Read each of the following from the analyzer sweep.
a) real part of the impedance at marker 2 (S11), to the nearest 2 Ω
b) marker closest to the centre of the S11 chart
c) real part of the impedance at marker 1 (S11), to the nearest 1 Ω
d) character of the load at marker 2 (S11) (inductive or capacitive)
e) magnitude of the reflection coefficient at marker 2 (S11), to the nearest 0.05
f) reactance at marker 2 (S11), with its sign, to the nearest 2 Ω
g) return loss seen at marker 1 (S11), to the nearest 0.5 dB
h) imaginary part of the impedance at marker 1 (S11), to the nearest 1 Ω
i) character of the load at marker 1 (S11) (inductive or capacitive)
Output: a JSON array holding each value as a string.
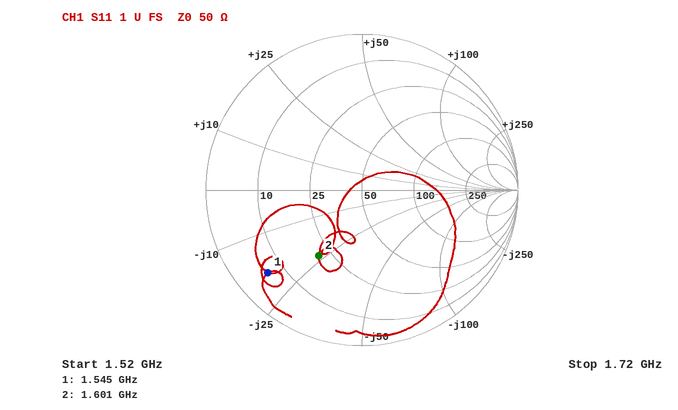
["20 Ω", "marker 2", "6 Ω", "capacitive", "0.50", "-24 Ω", "2.0 dB", "-19 Ω", "capacitive"]
